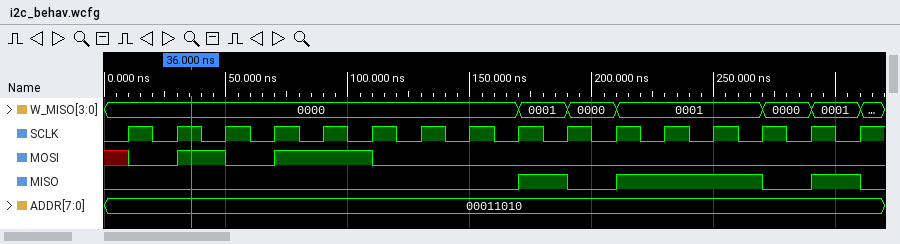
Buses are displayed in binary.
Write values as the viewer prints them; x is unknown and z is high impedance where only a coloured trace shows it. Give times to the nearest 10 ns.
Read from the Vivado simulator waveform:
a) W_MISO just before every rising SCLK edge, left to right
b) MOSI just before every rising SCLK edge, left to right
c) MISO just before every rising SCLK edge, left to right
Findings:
0000, 0000, 0000, 0000, 0000, 0000, 0000, 0000, 0000, 0001, 0000, 0001, 0001, 0001, 0000, 0001
x 0 1 0 1 1 0 0 0 0 0 0 0 0 0 0
0 0 0 0 0 0 0 0 0 1 0 1 1 1 0 1
